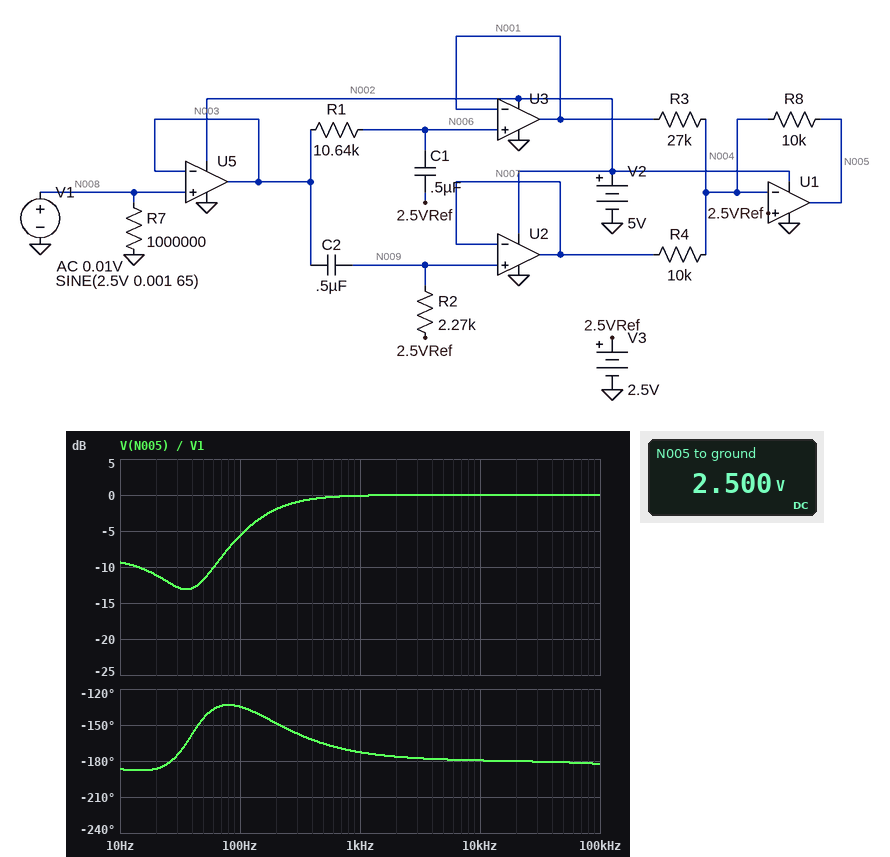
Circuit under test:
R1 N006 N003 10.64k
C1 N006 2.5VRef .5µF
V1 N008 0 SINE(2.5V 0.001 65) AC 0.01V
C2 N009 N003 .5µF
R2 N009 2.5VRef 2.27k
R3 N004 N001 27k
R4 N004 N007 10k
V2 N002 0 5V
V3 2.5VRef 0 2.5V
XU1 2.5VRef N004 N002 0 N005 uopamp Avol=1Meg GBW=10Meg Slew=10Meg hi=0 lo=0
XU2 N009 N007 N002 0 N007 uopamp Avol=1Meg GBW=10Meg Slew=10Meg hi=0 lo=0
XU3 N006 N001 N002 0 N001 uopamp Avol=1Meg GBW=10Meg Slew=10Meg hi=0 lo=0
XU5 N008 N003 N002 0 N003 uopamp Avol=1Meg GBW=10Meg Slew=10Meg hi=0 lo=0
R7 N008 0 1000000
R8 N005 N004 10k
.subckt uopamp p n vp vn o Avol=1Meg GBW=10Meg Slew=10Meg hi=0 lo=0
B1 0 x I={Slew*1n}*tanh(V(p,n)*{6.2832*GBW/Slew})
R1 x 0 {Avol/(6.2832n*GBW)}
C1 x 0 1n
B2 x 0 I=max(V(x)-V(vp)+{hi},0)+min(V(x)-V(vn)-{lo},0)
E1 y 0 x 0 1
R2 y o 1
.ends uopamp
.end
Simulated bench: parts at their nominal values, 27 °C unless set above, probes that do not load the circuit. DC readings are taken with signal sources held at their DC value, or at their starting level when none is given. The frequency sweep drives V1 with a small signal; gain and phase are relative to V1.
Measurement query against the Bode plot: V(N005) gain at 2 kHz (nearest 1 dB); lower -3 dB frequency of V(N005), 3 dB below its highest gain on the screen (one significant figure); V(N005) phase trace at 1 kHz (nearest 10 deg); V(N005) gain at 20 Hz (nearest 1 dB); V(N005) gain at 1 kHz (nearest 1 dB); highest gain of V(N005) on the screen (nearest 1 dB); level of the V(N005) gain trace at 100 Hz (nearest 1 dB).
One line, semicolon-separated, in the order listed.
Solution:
0 dB; 200 Hz; -170 deg; -11 dB; 0 dB; 0 dB; -6 dB
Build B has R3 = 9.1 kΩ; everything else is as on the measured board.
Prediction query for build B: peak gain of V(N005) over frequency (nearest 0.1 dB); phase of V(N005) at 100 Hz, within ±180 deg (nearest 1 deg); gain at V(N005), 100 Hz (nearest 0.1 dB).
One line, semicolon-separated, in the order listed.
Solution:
0.8 dB; -158 deg; -6.7 dB
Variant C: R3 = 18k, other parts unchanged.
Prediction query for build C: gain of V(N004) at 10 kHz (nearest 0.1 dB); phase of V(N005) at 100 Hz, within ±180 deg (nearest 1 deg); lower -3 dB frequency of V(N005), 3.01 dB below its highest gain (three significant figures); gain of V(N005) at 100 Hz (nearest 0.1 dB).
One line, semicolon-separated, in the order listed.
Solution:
-60.0 dB; -140 deg; 161 Hz; -6.0 dB
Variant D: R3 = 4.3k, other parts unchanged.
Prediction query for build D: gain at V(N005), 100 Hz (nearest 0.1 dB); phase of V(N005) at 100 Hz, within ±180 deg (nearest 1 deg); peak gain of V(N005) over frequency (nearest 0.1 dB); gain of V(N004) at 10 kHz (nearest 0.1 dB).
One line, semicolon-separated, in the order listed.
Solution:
-5.1 dB; 163 deg; 7.3 dB; -60.0 dB
